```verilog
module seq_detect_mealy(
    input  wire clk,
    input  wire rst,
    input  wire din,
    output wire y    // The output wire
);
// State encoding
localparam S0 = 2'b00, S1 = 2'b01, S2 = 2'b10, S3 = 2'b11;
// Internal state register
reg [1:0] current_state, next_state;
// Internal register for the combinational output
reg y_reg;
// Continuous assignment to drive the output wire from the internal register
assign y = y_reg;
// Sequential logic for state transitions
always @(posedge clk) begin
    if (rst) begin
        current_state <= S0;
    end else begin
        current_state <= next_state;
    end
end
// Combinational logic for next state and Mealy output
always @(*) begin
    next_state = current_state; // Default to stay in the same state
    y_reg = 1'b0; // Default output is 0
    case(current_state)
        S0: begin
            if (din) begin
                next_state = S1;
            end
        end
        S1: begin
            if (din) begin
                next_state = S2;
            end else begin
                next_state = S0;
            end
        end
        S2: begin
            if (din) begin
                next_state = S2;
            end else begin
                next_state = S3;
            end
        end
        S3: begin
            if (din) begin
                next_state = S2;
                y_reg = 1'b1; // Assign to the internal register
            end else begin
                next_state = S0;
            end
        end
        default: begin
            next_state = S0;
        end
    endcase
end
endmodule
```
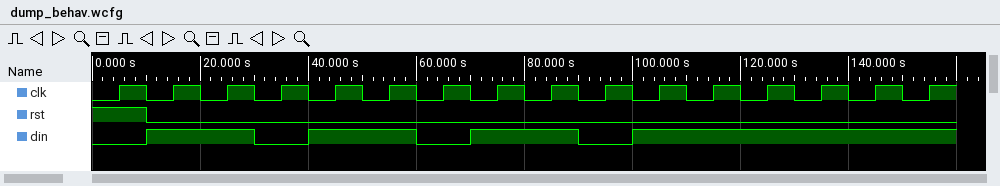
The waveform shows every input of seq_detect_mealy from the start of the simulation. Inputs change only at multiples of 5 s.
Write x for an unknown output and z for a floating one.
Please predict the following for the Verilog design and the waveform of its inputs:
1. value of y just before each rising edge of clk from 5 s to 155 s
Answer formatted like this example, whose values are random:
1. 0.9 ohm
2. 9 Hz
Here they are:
1. 0 0 0 0 1 0 0 1 0 0 1 0 0 0 0 0
